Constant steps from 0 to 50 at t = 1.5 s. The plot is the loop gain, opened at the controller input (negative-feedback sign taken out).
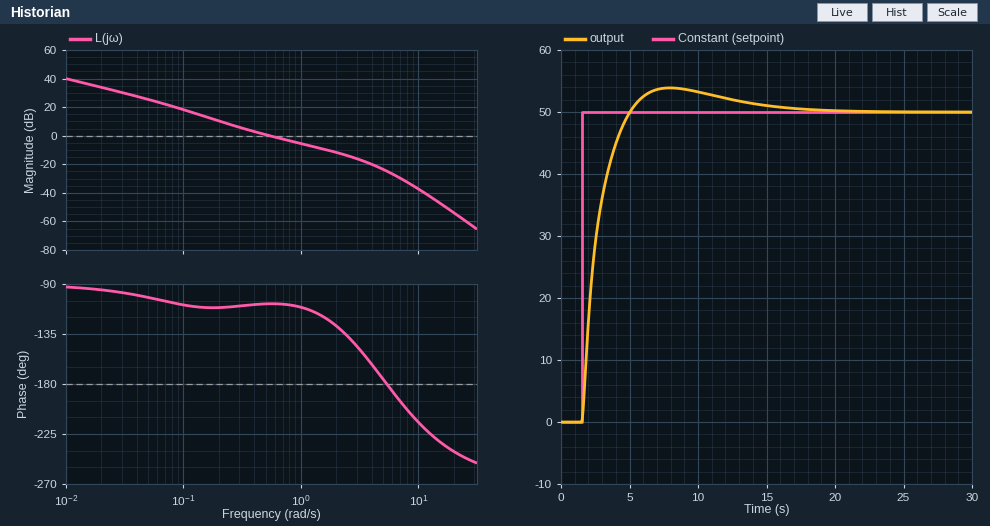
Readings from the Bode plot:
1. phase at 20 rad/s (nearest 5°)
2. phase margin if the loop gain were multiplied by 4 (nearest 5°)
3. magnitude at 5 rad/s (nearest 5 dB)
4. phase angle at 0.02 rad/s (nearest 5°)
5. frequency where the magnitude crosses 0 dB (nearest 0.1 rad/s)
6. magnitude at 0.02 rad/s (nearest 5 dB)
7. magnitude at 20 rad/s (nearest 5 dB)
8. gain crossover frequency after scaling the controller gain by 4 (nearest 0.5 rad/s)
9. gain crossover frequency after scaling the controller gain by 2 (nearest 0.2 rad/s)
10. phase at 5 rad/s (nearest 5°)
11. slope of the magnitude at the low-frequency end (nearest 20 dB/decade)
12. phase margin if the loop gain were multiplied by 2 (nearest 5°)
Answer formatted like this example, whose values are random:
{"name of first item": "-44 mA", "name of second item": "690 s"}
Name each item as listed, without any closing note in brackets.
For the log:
{"phase at 20 rad/s": "-240°", "phase margin if the loop gain were multiplied by 4": "50°", "magnitude at 5 rad/s": "-25 dB", "phase angle at 0.02 rad/s": "-95°", "frequency where the magnitude crosses 0 dB": "0.5 rad/s", "magnitude at 0.02 rad/s": "35 dB", "magnitude at 20 rad/s": "-55 dB", "gain crossover frequency after scaling the controller gain by 4": "2.0 rad/s", "gain crossover frequency after scaling the controller gain by 2": "1.0 rad/s", "phase at 5 rad/s": "-175°", "slope of the magnitude at the low-frequency end": "-20 dB/decade", "phase margin if the loop gain were multiplied by 2": "70°"}
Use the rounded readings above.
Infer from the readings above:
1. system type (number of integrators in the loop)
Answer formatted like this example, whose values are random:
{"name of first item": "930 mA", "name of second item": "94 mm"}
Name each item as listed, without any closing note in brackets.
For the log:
{"system type": "1"}
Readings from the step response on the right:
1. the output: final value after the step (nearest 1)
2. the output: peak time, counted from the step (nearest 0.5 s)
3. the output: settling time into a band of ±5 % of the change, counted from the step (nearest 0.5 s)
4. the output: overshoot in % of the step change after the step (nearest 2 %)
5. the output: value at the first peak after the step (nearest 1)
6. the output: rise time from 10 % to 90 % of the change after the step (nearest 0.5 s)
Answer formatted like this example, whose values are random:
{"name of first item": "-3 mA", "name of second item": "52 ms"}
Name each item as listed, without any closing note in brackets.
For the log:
{"the output: final value after the step": "50", "the output: peak time, counted from the step": "6.5 s", "the output: settling time into a band of ±5 % of the change, counted from the step": "10.0 s", "the output: overshoot in % of the step change after the step": "8 %", "the output: value at the first peak after the step": "54", "the output: rise time from 10 % to 90 % of the change after the step": "2.5 s"}
